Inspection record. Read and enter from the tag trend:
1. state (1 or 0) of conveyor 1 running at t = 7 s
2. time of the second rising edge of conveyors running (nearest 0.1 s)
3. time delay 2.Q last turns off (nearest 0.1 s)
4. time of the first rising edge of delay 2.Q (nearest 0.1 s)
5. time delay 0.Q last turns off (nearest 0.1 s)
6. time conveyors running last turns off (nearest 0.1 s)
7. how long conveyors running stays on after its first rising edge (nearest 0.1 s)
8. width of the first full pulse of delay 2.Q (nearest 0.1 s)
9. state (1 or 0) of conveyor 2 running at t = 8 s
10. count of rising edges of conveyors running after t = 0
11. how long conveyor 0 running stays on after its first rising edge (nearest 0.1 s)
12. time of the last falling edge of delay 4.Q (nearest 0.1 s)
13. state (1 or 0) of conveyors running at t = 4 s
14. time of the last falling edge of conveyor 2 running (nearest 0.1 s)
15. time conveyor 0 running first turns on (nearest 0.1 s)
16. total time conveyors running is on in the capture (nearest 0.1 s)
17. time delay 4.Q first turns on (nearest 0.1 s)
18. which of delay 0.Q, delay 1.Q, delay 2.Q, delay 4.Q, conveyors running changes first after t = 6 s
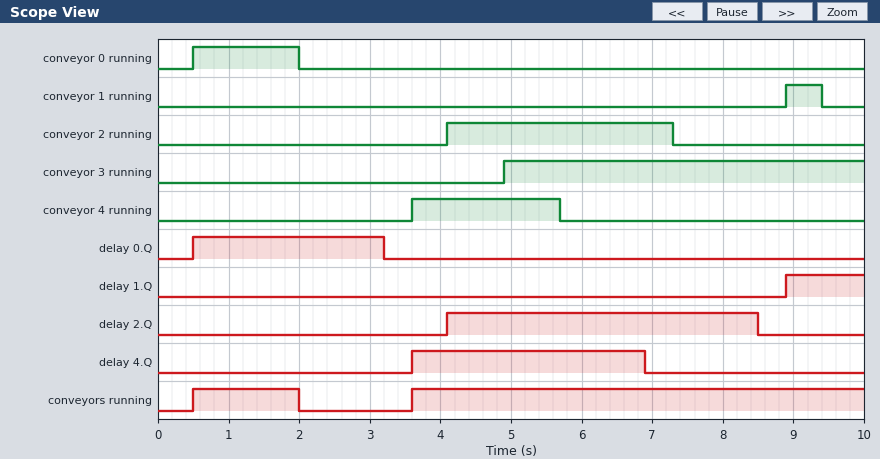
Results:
0
3.6 s
8.5 s
4.1 s
3.2 s
2.0 s
1.5 s
4.4 s
0
2
1.5 s
6.9 s
1
7.3 s
0.5 s
7.9 s
3.6 s
delay 4.Q
